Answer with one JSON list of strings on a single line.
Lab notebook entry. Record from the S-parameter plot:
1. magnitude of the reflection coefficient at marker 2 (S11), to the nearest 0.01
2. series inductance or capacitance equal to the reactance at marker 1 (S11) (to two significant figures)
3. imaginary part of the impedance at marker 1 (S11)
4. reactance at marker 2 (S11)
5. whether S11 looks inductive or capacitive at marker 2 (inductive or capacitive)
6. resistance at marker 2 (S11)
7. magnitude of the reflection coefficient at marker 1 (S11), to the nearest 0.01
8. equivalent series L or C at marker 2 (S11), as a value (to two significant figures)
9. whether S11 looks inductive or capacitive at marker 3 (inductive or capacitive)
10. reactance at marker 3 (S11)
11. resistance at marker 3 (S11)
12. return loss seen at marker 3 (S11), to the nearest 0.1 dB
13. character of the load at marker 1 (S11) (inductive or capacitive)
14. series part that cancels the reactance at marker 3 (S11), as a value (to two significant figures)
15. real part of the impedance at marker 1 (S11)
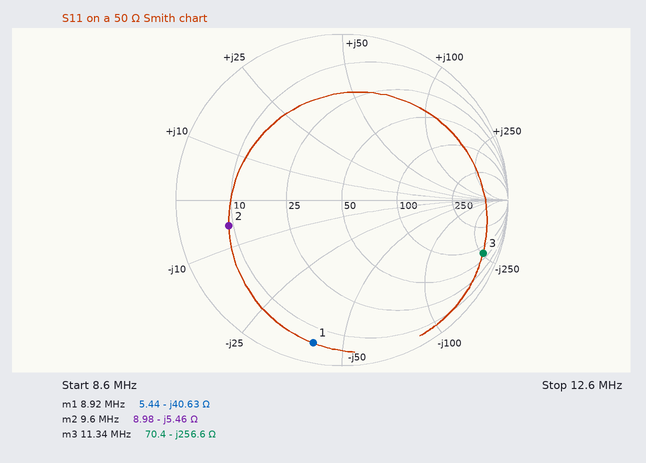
["0.70", "440 pF", "-40.63 Ω", "-5.46 Ω", "capacitive", "8.98 Ω", "0.88", "3.0 nF", "capacitive", "-256.6 Ω", "70.4 Ω", "0.8 dB", "capacitive", "3.6 µH", "5.44 Ω"]
